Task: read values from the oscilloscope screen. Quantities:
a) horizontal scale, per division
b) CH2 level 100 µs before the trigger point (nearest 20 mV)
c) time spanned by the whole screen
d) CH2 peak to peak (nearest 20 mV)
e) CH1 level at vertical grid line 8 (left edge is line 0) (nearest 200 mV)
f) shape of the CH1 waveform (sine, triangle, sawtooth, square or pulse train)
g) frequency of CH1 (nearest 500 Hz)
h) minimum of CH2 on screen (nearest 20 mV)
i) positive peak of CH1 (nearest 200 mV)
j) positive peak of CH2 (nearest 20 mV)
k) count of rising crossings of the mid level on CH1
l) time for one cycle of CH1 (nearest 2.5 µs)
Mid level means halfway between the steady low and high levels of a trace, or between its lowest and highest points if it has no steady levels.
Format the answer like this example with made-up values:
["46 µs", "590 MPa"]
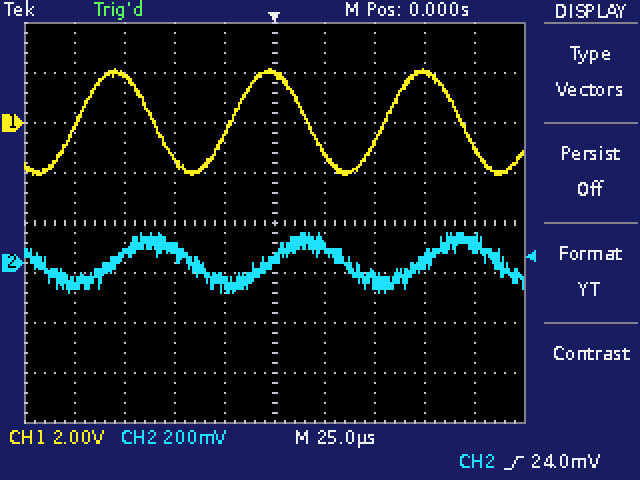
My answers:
["25 µs", "-80 mV", "250 µs", "240 mV", "2.0 V", "sine", "13.0 kHz", "-120 mV", "2.2 V", "120 mV", "3", "77.5 µs"]
